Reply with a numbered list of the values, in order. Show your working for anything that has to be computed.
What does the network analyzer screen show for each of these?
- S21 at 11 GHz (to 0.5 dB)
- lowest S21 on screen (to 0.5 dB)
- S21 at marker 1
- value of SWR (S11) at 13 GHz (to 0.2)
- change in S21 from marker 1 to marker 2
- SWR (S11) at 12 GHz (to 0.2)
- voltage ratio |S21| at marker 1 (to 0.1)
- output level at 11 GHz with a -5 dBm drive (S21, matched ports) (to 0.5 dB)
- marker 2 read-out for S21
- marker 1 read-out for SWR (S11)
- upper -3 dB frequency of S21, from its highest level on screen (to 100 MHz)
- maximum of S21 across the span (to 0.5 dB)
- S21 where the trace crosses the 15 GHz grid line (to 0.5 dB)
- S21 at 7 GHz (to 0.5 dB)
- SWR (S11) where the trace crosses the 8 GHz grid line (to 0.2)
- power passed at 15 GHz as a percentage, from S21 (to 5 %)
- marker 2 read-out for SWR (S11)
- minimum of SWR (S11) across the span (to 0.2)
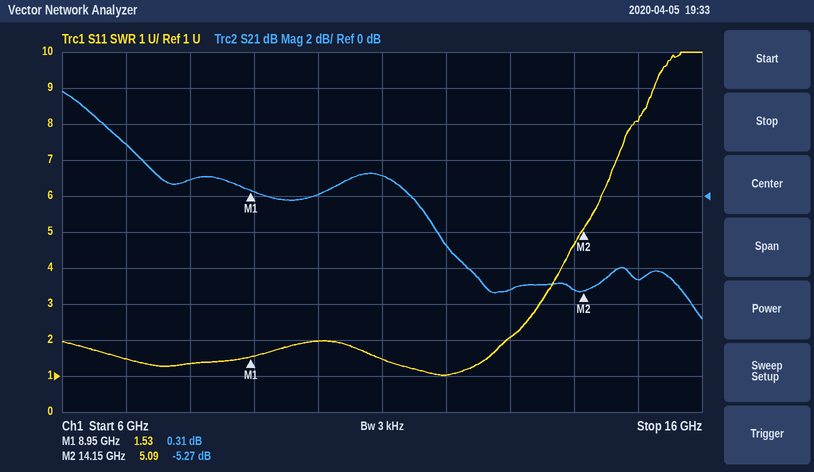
1. 1.0 dB
2. -7.0 dB
3. 0.31 dB
4. 2.0
5. -5.27 − (0.31) = -5.58 dB
6. 1.0
7. 10^(0.31/20) ≈ 1.0
8. -5 dBm + (1.0 dB) = -4.0 dBm
9. -5.27 dB
10. 1.53
11. 7.0 GHz
12. 6.0 dB
13. -4.5 dB
14. 3.0 dB
15. 1.4
16. 10^(-4.5/10) ≈ 35 %
17. 5.09
18. 1.0
